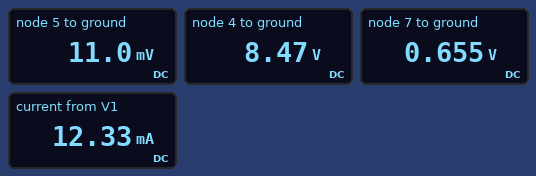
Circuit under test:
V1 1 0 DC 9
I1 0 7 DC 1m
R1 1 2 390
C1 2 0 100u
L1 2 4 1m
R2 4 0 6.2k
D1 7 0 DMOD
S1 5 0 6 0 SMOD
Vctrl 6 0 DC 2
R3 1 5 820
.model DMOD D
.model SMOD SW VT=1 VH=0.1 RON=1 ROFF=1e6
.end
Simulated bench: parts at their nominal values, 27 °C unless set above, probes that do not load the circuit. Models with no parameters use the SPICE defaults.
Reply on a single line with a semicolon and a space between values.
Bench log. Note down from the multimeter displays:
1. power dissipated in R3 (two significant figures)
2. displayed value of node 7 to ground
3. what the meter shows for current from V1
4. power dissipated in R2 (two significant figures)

99 mW; 0.655 V; 12.33 mA; 12 mW
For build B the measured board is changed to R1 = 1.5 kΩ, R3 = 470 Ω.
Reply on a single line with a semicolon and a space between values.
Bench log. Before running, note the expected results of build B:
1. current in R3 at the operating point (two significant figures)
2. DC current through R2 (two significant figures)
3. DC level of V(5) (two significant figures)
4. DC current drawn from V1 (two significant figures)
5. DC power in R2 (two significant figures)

19 mA; 1.2 mA; 19 mV; 20 mA; 8.5 mW
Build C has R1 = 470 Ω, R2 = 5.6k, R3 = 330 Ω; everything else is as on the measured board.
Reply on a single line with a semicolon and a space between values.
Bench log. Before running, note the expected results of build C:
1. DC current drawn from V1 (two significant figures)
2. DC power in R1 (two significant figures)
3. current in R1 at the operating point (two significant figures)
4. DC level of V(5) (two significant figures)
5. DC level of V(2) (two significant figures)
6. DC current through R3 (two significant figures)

29 mA; 1.0 mW; 1.5 mA; 27 mV; 8.3 V; 27 mA
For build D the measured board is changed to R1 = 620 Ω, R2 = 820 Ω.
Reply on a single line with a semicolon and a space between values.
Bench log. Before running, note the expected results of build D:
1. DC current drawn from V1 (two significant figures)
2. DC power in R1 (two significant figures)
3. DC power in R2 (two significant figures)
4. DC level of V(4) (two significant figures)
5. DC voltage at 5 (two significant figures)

17 mA; 24 mW; 32 mW; 5.1 V; 11 mV
